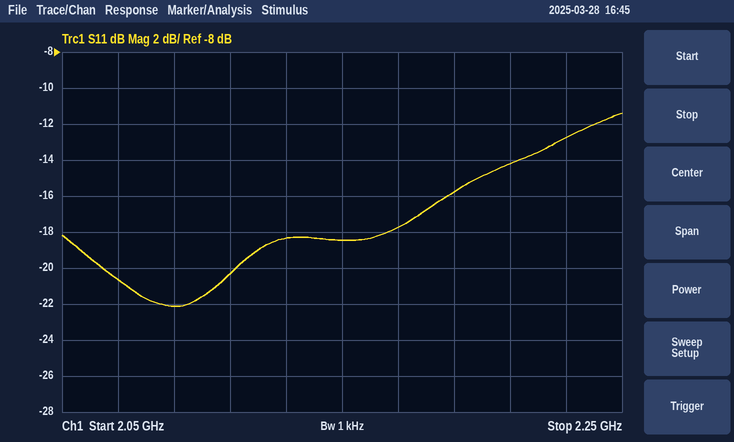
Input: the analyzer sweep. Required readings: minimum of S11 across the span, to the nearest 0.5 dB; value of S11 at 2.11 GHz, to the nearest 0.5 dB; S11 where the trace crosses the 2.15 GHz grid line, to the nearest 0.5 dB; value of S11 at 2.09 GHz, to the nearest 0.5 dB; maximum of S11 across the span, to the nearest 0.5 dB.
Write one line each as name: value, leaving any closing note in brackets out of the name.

minimum of S11 across the span, to the nearest 0.5 dB: -22.0 dB
value of S11 at 2.11 GHz, to the nearest 0.5 dB: -20.5 dB
S11 where the trace crosses the 2.15 GHz grid line, to the nearest 0.5 dB: -18.5 dB
value of S11 at 2.09 GHz, to the nearest 0.5 dB: -22.0 dB
maximum of S11 across the span, to the nearest 0.5 dB: -11.5 dB
